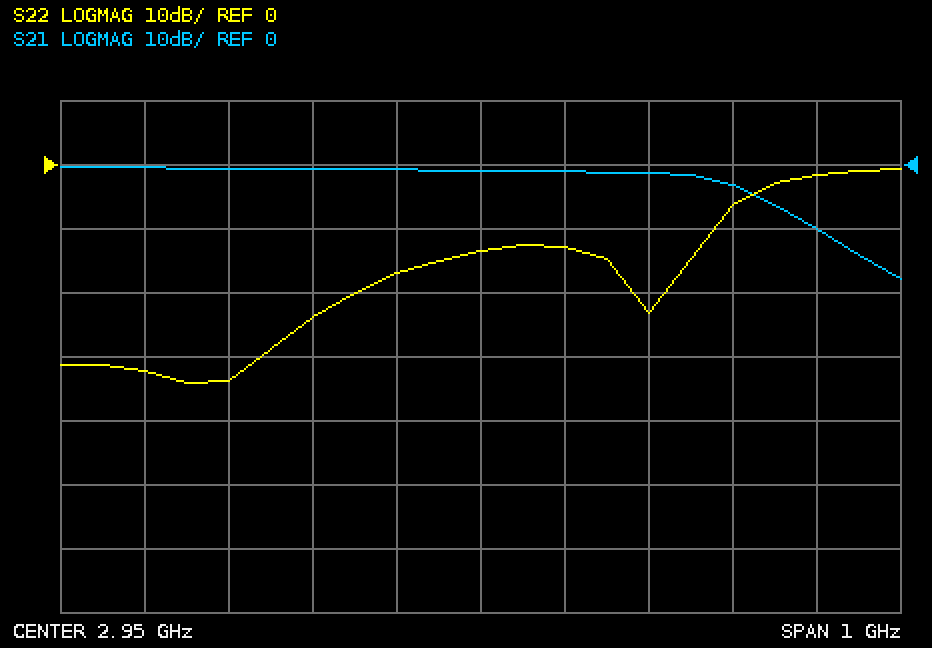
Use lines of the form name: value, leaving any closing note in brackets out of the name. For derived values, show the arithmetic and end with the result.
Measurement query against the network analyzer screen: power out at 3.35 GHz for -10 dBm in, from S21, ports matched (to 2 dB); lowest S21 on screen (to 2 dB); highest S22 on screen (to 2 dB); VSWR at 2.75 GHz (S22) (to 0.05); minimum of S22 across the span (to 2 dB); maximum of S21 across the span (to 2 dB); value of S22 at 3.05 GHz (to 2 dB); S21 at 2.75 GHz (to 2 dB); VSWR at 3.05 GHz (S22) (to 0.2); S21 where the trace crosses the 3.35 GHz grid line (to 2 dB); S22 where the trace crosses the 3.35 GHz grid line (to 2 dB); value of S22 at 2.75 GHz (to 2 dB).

power out at 3.35 GHz for -10 dBm in, from S21, ports matched: -10 dBm + (-10 dB) = -20 dBm
lowest S21 on screen: -18 dB
highest S22 on screen: 0 dB
VSWR at 2.75 GHz (S22): |Γ| = 10^(-24/20) = 0.0631; VSWR = (1 + 0.0631)/(1 − 0.0631) ≈ 1.13, so 1.15 to the nearest 0.05
minimum of S22 across the span: -34 dB
maximum of S21 across the span: 0 dB
value of S22 at 3.05 GHz: -12 dB
S21 at 2.75 GHz: 0 dB
VSWR at 3.05 GHz (S22): |Γ| = 10^(-12/20) = 0.2512; VSWR = (1 + 0.2512)/(1 − 0.2512) ≈ 1.67, so 1.6 to the nearest 0.2
S21 where the trace crosses the 3.35 GHz grid line: -10 dB
S22 where the trace crosses the 3.35 GHz grid line: -2 dB
value of S22 at 2.75 GHz: -24 dB
